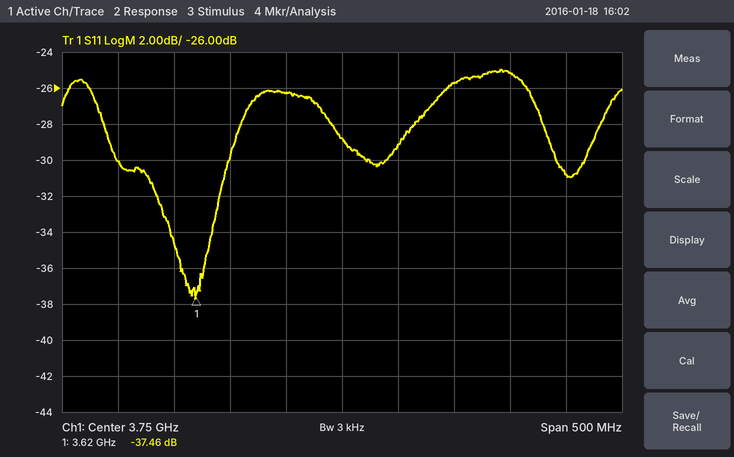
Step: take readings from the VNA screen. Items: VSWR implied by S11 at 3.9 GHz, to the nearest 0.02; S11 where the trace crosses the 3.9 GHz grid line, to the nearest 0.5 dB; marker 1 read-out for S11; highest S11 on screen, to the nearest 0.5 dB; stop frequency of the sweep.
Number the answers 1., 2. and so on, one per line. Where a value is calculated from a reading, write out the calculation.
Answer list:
1. |Γ| = 10^(-25/20) = 0.0562; VSWR = (1 + 0.0562)/(1 − 0.0562) ≈ 1.12
2. -25.0 dB
3. -37.46 dB
4. -25.0 dB
5. 4 GHz
